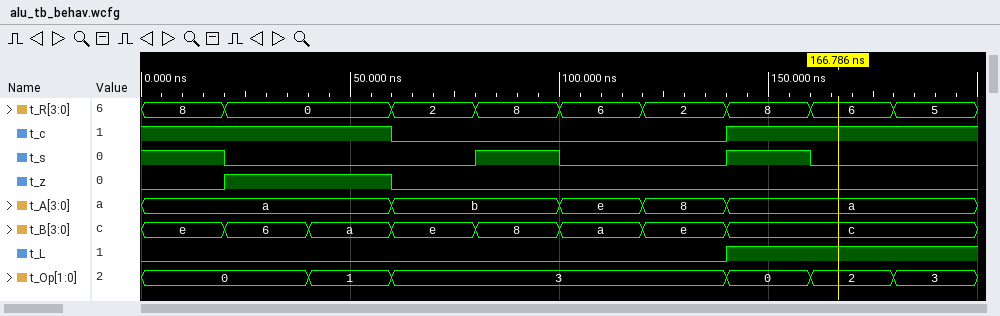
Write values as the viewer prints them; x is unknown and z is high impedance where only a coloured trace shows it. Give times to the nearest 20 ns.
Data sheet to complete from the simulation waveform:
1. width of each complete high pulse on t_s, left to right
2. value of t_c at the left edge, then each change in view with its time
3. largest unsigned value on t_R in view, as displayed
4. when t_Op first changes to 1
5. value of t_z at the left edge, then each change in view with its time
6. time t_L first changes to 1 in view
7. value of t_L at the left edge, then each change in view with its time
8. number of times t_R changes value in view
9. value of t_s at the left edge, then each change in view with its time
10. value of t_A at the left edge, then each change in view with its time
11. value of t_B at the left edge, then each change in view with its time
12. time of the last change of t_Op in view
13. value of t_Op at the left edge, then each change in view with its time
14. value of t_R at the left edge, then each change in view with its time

20 ns, 20 ns
1, 0 at 60 ns, 1 at 140 ns
8
40 ns
0, 1 at 20 ns, 0 at 60 ns
140 ns
0, 1 at 140 ns
8
1, 0 at 20 ns, 1 at 80 ns, 0 at 100 ns, 1 at 140 ns, 0 at 160 ns
a, b at 60 ns, e at 100 ns, 8 at 120 ns, a at 140 ns
e, 6 at 20 ns, a at 40 ns, e at 60 ns, 8 at 80 ns, a at 100 ns, e at 120 ns, c at 140 ns
180 ns
0, 1 at 40 ns, 3 at 60 ns, 0 at 140 ns, 2 at 160 ns, 3 at 180 ns
8, 0 at 20 ns, 2 at 60 ns, 8 at 80 ns, 6 at 100 ns, 2 at 120 ns, 8 at 140 ns, 6 at 160 ns, 5 at 180 ns
